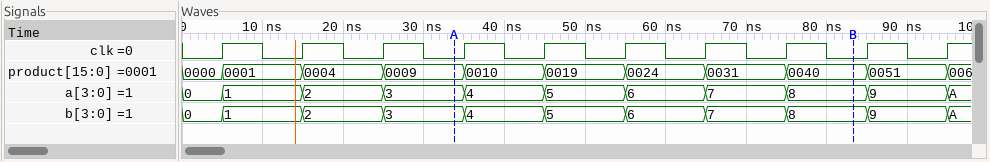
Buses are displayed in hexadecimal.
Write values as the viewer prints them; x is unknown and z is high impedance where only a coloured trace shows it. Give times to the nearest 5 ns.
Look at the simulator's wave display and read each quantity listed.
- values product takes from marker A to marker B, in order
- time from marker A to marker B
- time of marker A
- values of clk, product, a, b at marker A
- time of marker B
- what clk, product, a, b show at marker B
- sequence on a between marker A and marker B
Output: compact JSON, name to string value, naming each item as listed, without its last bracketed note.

{"values product takes from marker A to marker B, in order": "0009, 0010, 0019, 0024, 0031, 0040", "time from marker A to marker B": "50 ns", "time of marker A": "35 ns", "values of clk, product, a, b at marker A": "clk=0, product=0009, a=3, b=3", "time of marker B": "85 ns", "what clk, product, a, b show at marker B": "clk=0, product=0040, a=8, b=8", "sequence on a between marker A and marker B": "3, 4, 5, 6, 7, 8"}
